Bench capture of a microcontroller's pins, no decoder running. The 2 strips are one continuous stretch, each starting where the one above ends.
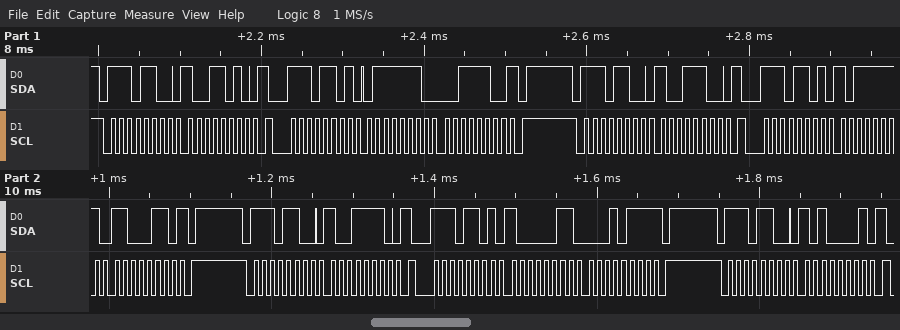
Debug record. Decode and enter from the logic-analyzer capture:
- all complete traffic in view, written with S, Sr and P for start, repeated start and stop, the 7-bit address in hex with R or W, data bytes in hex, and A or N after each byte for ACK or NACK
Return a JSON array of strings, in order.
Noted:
["S 76W A 9A A Sr 76R A 7E A 3C N P S 76W A 9C A Sr 76R A BF A C6 N P S 76W A 9E A Sr 76R A 83 A 17 N P S 76W A A1 A"]
